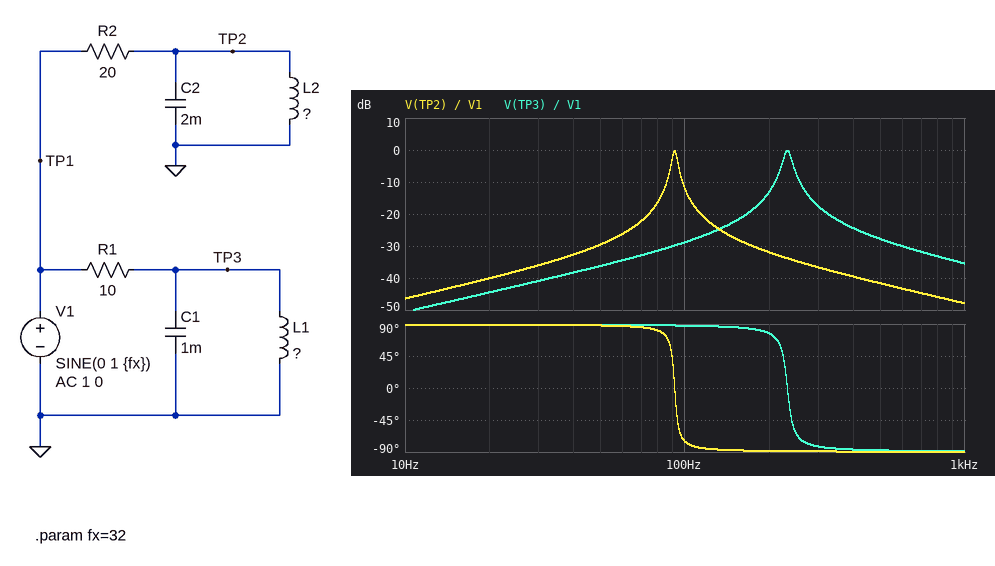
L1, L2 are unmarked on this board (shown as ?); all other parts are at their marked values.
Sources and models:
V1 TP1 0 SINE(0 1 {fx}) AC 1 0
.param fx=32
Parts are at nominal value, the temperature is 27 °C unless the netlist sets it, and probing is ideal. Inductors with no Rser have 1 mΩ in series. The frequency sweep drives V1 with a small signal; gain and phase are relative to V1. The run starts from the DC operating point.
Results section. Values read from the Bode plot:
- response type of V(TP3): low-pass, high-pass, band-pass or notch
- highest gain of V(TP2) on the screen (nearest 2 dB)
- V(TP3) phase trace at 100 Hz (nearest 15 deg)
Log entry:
band-pass
0 dB
90 deg
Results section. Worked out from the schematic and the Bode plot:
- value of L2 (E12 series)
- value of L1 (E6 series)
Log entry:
1.5 mH
470 µH
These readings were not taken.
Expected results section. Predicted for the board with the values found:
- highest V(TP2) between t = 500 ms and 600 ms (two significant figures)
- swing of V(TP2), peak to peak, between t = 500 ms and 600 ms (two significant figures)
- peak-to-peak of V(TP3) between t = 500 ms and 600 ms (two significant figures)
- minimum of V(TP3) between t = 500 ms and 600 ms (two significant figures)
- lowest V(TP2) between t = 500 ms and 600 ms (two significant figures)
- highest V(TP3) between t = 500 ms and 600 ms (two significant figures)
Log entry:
17 mV
34 mV
19 mV
-9.6 mV
-17 mV
9.6 mV
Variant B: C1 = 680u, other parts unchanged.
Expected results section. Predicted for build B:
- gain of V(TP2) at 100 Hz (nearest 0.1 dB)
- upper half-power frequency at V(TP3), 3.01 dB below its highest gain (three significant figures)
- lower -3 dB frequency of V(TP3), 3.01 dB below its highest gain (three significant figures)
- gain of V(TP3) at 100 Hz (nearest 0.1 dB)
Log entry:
-12.1 dB
294 Hz
270 Hz
-29.4 dB
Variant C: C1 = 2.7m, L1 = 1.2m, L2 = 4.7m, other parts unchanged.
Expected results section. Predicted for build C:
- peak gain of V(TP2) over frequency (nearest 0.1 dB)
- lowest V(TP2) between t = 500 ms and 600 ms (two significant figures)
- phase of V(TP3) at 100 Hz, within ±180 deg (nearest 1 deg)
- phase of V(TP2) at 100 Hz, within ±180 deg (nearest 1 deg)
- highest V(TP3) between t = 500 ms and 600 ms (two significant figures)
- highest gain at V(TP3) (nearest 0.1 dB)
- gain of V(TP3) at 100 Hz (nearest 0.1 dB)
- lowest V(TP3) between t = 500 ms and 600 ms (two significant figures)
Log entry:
-0.1 dB
-76 mV
-75 deg
-87 deg
28 mV
-0.2 dB
-11.7 dB
-28 mV
